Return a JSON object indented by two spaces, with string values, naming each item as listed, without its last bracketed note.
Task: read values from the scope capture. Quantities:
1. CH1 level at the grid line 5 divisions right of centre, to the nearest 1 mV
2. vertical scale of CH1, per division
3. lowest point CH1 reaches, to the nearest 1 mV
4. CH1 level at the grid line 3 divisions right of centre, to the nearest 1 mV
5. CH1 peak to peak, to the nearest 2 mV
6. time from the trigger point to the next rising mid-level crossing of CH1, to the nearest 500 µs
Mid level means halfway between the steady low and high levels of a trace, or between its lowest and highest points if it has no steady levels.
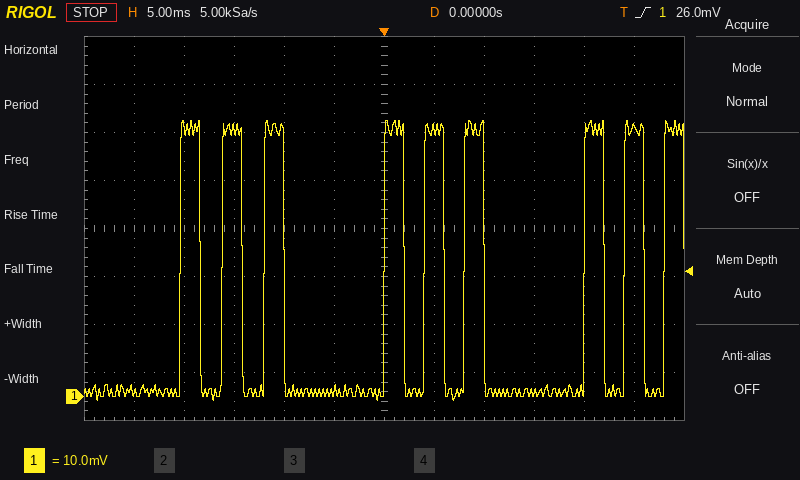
{
  "CH1 level at the grid line 5 divisions right of centre, to the nearest 1 mV": "56 mV",
  "vertical scale of CH1, per division": "10 mV",
  "lowest point CH1 reaches, to the nearest 1 mV": "-1 mV",
  "CH1 level at the grid line 3 divisions right of centre, to the nearest 1 mV": "1 mV",
  "CH1 peak to peak, to the nearest 2 mV": "58 mV",
  "time from the trigger point to the next rising mid-level crossing of CH1, to the nearest 500 µs": "4.0 ms"
}
